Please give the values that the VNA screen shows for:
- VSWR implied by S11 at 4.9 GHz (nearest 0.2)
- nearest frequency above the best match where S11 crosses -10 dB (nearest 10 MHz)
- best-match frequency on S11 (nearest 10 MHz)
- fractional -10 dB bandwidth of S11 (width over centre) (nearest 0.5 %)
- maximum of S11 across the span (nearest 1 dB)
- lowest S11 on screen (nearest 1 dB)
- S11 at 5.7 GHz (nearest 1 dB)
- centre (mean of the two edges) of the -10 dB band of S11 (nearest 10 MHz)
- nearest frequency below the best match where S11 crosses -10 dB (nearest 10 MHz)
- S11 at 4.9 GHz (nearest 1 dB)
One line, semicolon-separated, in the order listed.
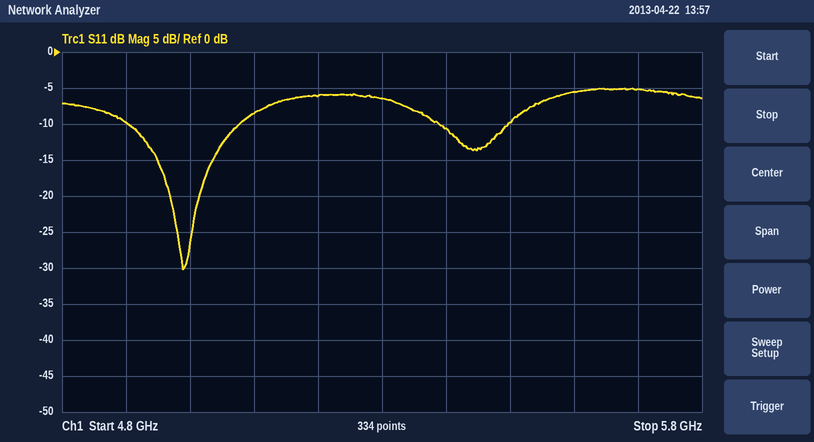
2.0; 5.08 GHz; 4.99 GHz; 3.5 %; -5 dB; -30 dB; -5 dB; 4.99 GHz; 4.90 GHz; -10 dB
